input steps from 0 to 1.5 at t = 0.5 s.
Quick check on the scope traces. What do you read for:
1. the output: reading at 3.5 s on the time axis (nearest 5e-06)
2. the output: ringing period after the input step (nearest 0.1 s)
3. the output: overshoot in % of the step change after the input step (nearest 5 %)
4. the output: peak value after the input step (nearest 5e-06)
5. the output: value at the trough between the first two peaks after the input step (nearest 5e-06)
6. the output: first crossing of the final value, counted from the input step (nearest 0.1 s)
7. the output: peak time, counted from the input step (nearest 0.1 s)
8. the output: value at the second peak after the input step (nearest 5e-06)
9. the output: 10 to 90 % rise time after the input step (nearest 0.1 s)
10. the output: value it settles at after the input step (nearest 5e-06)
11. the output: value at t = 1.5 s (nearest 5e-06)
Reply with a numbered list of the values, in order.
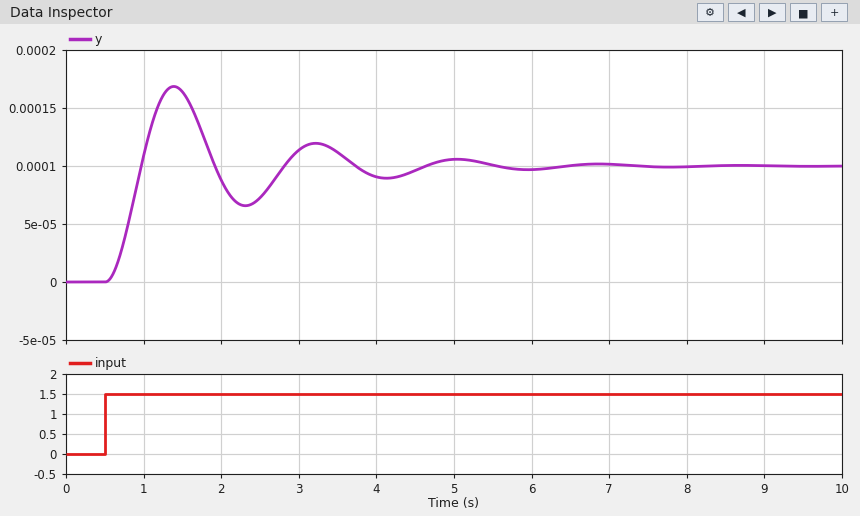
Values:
1. 0.000110
2. 1.8 s
3. 70 %
4. 0.000170
5. 0.000065
6. 0.5 s
7. 0.9 s
8. 0.000120
9. 0.3 s
10. 0.000100
11. 0.000165
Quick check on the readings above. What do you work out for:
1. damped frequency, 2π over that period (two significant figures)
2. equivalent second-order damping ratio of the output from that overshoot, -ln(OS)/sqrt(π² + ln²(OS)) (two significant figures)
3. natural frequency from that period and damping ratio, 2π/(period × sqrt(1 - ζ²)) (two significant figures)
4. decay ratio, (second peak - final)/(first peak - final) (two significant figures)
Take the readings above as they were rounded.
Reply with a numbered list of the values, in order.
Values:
1. 3.5 rad/s
2. 0.11
3. 3.5 rad/s
4. 0.29
